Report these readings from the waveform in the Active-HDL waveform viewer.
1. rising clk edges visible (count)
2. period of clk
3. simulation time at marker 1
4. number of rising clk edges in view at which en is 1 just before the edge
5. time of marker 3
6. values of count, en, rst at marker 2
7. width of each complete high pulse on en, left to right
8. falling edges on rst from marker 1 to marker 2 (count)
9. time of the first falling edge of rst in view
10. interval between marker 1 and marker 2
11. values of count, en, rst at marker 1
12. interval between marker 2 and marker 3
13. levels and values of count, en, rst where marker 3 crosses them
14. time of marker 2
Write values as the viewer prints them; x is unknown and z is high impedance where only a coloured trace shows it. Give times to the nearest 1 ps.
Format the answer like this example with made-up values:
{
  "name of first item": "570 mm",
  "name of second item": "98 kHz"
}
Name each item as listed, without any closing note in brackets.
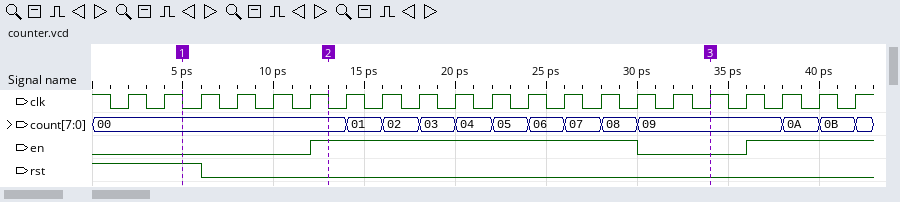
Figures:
{
  "rising clk edges visible": "21",
  "period of clk": "2 ps",
  "simulation time at marker 1": "5 ps",
  "number of rising clk edges in view at which en is 1 just before the edge": "12",
  "time of marker 3": "34 ps",
  "values of count, en, rst at marker 2": "count=00, en=1, rst=0",
  "width of each complete high pulse on en, left to right": "18 ps",
  "falling edges on rst from marker 1 to marker 2": "1",
  "time of the first falling edge of rst in view": "6 ps",
  "interval between marker 1 and marker 2": "8 ps",
  "values of count, en, rst at marker 1": "count=00, en=0, rst=1",
  "interval between marker 2 and marker 3": "21 ps",
  "levels and values of count, en, rst where marker 3 crosses them": "count=09, en=0, rst=0",
  "time of marker 2": "13 ps"
}
